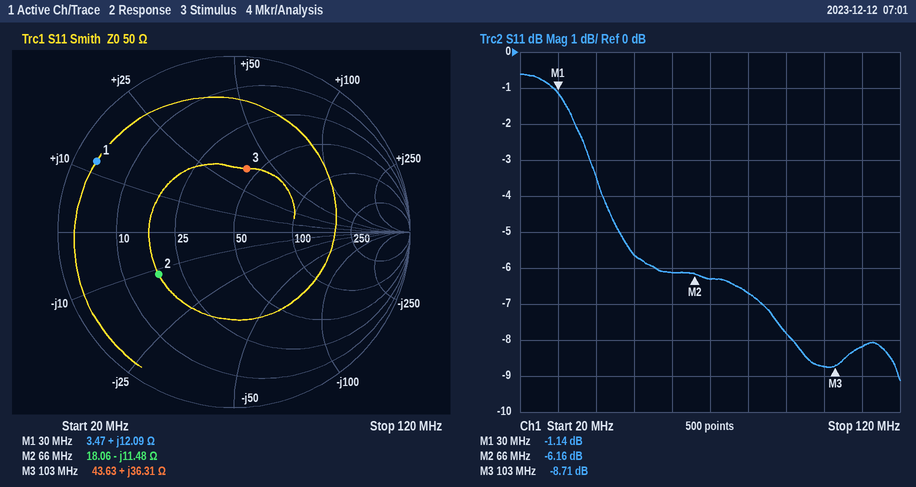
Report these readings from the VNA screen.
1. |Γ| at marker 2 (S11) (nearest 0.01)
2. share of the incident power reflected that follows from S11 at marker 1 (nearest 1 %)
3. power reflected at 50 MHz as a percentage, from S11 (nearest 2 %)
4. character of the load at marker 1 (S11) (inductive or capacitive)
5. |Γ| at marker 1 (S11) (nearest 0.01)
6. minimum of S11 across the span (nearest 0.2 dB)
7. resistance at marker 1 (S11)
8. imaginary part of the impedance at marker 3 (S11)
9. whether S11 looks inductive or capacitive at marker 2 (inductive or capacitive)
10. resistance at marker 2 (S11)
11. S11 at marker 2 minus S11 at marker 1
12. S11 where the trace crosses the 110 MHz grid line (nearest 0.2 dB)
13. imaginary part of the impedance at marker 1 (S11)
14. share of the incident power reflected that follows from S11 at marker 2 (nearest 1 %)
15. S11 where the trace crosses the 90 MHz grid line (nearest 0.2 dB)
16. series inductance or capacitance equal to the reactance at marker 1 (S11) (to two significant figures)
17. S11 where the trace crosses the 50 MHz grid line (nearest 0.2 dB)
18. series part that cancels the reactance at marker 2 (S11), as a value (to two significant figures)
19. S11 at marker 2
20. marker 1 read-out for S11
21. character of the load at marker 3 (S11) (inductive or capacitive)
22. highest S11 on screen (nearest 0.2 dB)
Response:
0.49
77 %
28 %
inductive
0.88
-9.2 dB
3.47 Ω
+36.31 Ω
capacitive
18.06 Ω
-5.02 dB
-8.2 dB
+12.09 Ω
24 %
-7.8 dB
64 nH
-5.6 dB
28 nH
-6.16 dB
-1.14 dB
inductive
-0.6 dB
